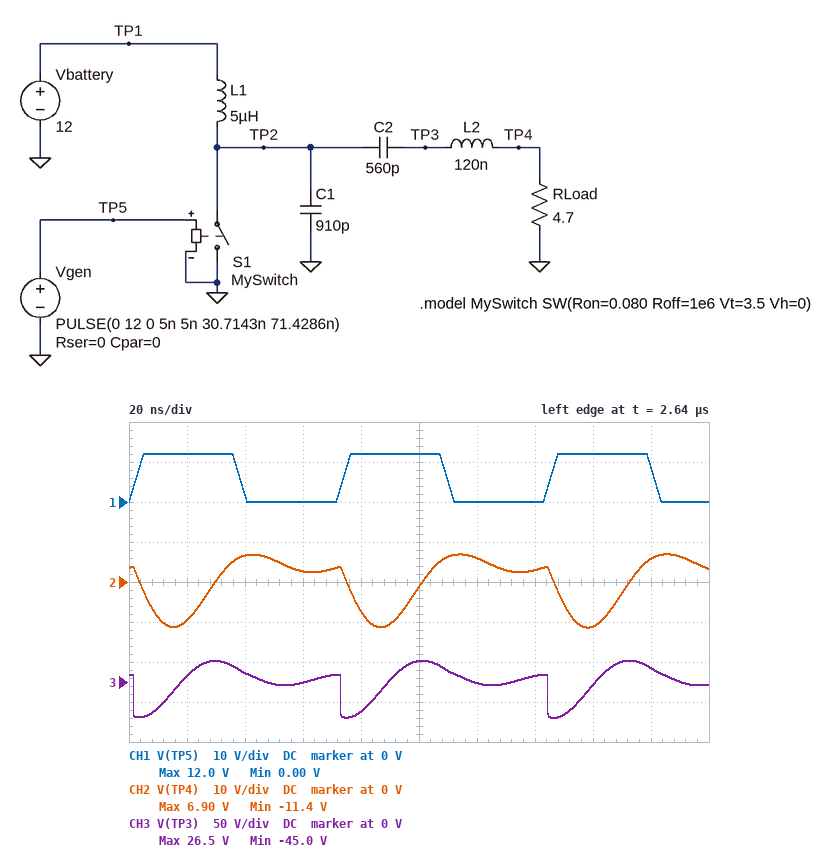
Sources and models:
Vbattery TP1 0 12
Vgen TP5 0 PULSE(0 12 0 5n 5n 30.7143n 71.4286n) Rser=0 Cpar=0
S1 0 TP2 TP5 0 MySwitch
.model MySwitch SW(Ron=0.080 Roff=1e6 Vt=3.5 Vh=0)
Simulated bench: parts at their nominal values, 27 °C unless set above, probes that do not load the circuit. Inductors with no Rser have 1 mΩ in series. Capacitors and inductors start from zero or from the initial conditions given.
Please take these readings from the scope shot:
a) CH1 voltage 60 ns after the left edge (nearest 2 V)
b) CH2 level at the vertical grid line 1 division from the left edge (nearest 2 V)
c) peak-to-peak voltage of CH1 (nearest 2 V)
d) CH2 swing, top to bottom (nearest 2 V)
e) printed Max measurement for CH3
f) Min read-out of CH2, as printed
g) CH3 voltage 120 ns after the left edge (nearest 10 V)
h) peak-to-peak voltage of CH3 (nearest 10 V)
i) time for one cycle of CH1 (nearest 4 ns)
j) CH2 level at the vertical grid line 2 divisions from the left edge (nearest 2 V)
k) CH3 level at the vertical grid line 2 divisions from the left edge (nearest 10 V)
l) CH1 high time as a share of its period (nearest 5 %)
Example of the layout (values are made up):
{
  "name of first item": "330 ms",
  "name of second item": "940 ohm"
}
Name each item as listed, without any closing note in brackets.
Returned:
{
  "CH1 voltage 60 ns after the left edge": "0 V",
  "CH2 level at the vertical grid line 1 division from the left edge": "-10 V",
  "peak-to-peak voltage of CH1": "12 V",
  "CH2 swing, top to bottom": "18 V",
  "printed Max measurement for CH3": "26.5 V",
  "Min read-out of CH2, as printed": "-11.4 V",
  "CH3 voltage 120 ns after the left edge": "0 V",
  "peak-to-peak voltage of CH3": "70 V",
  "time for one cycle of CH1": "72 ns",
  "CH2 level at the vertical grid line 2 divisions from the left edge": "6 V",
  "CH3 level at the vertical grid line 2 divisions from the left edge": "10 V",
  "CH1 high time as a share of its period": "50 %"
}
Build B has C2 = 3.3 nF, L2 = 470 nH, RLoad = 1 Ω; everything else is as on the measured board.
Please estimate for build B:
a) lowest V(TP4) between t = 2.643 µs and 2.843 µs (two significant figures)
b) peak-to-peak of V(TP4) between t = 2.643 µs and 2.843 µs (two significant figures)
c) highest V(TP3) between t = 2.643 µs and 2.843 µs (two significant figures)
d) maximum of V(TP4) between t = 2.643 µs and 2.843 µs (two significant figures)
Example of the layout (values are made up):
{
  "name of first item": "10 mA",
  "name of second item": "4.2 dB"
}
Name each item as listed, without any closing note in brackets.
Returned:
{
  "lowest V(TP4) between t = 2.643 µs and 2.843 µs": "-480 mV",
  "peak-to-peak of V(TP4) between t = 2.643 µs and 2.843 µs": "1.1 V",
  "highest V(TP3) between t = 2.643 µs and 2.843 µs": "32 V",
  "maximum of V(TP4) between t = 2.643 µs and 2.843 µs": "650 mV"
}
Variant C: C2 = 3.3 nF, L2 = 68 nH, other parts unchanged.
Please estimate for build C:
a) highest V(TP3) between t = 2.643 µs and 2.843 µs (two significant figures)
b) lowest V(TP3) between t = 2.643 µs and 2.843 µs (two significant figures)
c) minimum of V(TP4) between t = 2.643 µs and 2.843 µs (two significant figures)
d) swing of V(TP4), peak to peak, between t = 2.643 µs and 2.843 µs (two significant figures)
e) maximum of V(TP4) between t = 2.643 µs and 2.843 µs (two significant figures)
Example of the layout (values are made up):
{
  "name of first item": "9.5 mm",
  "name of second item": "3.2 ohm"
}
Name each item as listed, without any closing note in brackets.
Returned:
{
  "highest V(TP3) between t = 2.643 µs and 2.843 µs": "31 V",
  "lowest V(TP3) between t = 2.643 µs and 2.843 µs": "-22 V",
  "minimum of V(TP4) between t = 2.643 µs and 2.843 µs": "-12 V",
  "swing of V(TP4), peak to peak, between t = 2.643 µs and 2.843 µs": "28 V",
  "maximum of V(TP4) between t = 2.643 µs and 2.843 µs": "16 V"
}
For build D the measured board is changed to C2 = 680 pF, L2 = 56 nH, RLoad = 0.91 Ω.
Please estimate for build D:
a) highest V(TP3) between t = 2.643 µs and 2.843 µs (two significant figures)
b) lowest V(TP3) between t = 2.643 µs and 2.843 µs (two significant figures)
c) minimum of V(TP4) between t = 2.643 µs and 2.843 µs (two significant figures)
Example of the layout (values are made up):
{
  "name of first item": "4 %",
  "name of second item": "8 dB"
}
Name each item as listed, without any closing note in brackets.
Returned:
{
  "highest V(TP3) between t = 2.643 µs and 2.843 µs": "37 V",
  "lowest V(TP3) between t = 2.643 µs and 2.843 µs": "-41 V",
  "minimum of V(TP4) between t = 2.643 µs and 2.843 µs": "-4.1 V"
}
